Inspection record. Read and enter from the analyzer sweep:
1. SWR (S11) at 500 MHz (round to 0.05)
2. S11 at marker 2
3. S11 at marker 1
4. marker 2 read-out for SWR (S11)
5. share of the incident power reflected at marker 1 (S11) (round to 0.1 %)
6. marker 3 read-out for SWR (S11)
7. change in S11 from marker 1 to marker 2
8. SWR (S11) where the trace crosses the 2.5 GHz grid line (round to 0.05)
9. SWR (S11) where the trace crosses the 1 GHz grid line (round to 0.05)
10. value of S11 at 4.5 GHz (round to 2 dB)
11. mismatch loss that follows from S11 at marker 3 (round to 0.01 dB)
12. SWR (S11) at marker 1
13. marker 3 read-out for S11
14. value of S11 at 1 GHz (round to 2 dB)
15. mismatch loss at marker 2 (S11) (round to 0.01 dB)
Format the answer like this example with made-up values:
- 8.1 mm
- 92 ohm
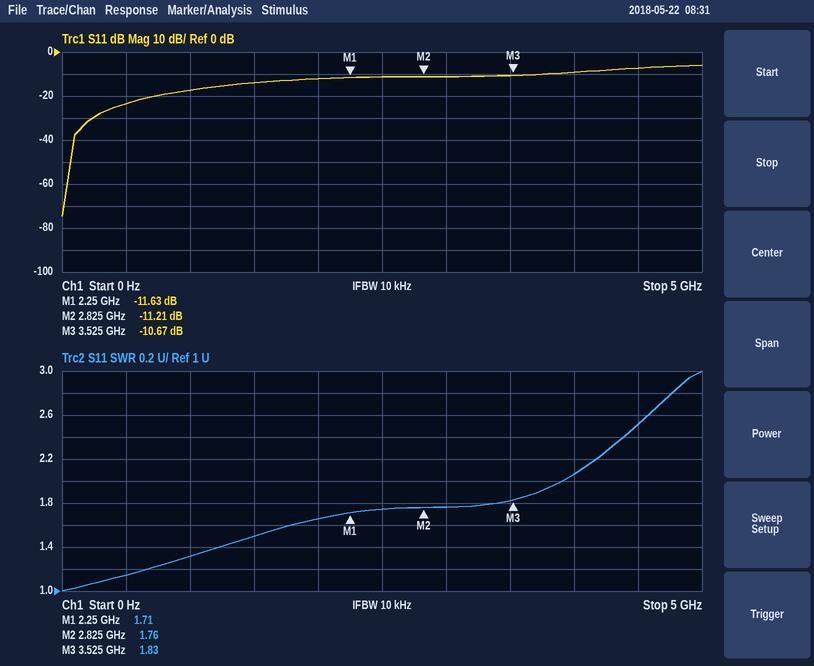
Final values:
- 1.15
- -11.21 dB
- -11.63 dB
- 1.76
- 6.9 %
- 1.83
- 0.42 dB
- 1.75
- 1.30
- -8 dB
- 0.39 dB
- 1.71
- -10.67 dB
- -18 dB
- 0.34 dB
